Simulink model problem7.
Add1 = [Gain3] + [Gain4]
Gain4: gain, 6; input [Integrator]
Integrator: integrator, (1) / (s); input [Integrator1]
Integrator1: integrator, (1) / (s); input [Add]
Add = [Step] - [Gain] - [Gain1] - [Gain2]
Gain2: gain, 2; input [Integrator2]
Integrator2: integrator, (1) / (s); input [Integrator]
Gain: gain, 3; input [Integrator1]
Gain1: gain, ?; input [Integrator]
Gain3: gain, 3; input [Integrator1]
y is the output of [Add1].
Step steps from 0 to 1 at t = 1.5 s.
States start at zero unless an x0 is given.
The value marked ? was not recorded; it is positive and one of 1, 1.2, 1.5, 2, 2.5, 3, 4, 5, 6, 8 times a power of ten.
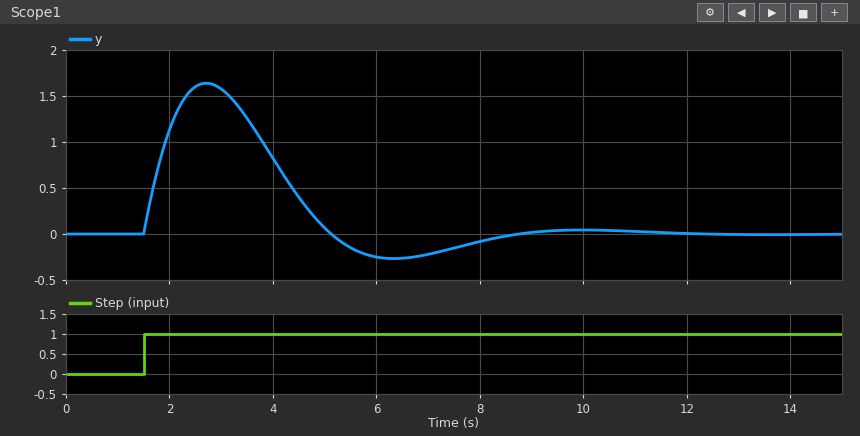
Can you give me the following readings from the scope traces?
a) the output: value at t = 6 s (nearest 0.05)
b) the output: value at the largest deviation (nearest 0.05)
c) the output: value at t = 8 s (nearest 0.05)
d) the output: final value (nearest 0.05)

-0.25
1.65
-0.10
0.00
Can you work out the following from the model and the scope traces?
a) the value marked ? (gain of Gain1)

3
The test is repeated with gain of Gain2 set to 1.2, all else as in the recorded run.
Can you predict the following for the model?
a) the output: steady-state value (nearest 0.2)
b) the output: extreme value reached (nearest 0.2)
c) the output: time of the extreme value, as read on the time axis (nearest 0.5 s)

0.0
1.8
3.0 s
